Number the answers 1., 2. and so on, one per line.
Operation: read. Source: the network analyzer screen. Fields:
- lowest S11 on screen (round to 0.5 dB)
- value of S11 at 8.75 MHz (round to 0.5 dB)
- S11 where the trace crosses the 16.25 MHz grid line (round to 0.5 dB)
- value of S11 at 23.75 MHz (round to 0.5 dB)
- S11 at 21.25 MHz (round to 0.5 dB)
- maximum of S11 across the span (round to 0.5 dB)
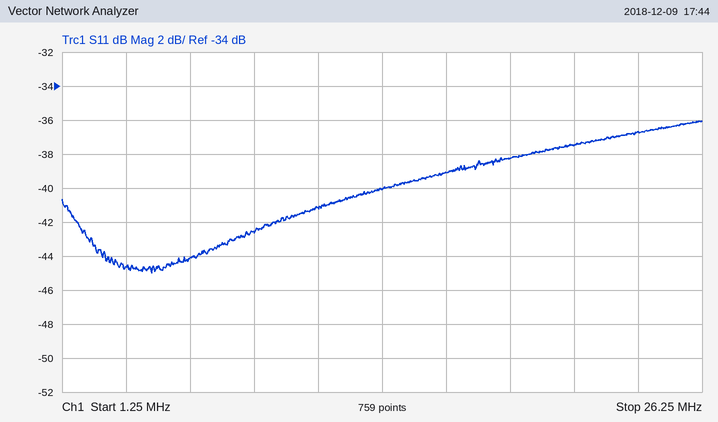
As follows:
1. -45.0 dB
2. -42.5 dB
3. -39.0 dB
4. -36.5 dB
5. -37.5 dB
6. -36.0 dB
